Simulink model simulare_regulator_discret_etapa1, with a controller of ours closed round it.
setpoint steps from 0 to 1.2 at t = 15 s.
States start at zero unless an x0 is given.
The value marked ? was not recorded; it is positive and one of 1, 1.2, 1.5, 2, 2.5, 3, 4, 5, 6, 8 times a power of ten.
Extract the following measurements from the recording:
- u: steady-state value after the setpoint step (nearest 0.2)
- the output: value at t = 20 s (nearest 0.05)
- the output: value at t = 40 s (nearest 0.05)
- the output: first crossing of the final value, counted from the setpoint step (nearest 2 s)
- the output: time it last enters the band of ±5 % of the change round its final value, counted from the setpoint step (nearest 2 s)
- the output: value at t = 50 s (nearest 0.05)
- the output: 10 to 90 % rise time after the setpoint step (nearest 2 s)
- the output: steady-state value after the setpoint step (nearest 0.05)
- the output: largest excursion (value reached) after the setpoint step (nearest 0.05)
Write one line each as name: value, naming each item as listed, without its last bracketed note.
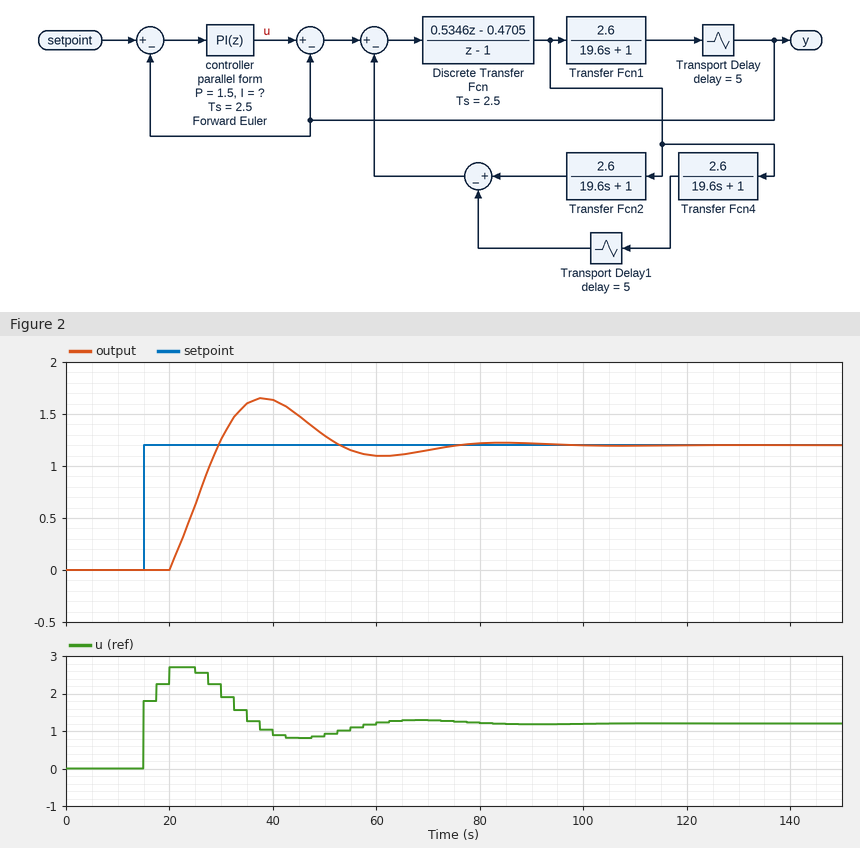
u: steady-state value after the setpoint step: 1.2
the output: value at t = 20 s: 0.00
the output: value at t = 40 s: 1.65
the output: first crossing of the final value, counted from the setpoint step: 14 s
the output: time it last enters the band of ±5 % of the change round its final value, counted from the setpoint step: 54 s
the output: value at t = 50 s: 1.30
the output: 10 to 90 % rise time after the setpoint step: 8 s
the output: steady-state value after the setpoint step: 1.20
the output: largest excursion (value reached) after the setpoint step: 1.65
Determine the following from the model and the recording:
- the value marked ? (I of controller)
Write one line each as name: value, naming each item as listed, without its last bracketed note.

the value marked ?: 0.15
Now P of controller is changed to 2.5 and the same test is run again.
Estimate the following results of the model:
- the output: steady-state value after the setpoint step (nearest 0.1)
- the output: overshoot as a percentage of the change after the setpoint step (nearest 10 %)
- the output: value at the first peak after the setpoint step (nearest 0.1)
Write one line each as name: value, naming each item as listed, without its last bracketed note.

the output: steady-state value after the setpoint step: 1.2
the output: overshoot as a percentage of the change after the setpoint step: 50 %
the output: value at the first peak after the setpoint step: 1.8
